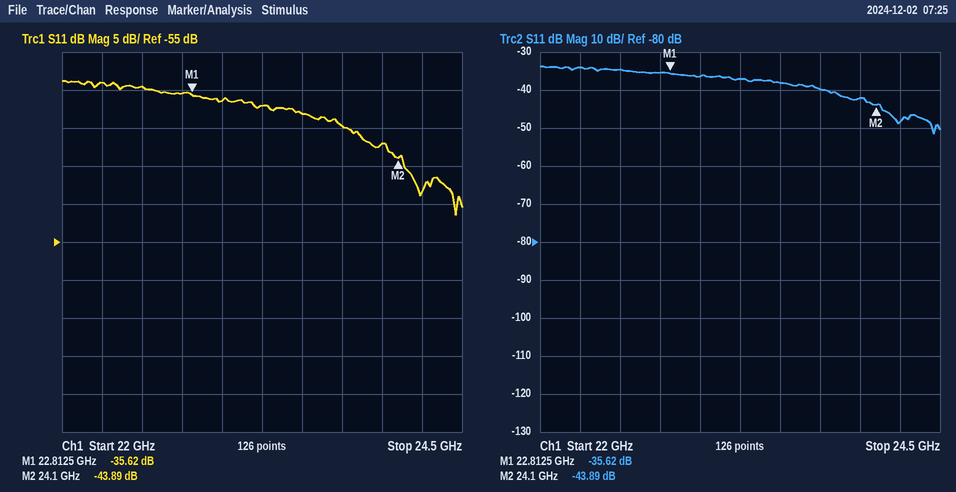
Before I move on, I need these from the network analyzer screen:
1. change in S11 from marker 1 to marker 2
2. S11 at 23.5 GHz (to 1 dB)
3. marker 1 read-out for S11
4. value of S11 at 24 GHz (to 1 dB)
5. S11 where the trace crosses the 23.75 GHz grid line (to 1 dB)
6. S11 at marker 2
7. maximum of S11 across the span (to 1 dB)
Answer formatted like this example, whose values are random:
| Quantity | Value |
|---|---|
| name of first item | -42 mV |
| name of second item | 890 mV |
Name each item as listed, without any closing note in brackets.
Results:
| Quantity | Value |
|---|---|
| change in S11 from marker 1 to marker 2 | -8.27 dB |
| S11 at 23.5 GHz | -38 dB |
| marker 1 read-out for S11 | -35.62 dB |
| value of S11 at 24 GHz | -42 dB |
| S11 where the trace crosses the 23.75 GHz grid line | -40 dB |
| S11 at marker 2 | -43.89 dB |
| maximum of S11 across the span | -34 dB |
